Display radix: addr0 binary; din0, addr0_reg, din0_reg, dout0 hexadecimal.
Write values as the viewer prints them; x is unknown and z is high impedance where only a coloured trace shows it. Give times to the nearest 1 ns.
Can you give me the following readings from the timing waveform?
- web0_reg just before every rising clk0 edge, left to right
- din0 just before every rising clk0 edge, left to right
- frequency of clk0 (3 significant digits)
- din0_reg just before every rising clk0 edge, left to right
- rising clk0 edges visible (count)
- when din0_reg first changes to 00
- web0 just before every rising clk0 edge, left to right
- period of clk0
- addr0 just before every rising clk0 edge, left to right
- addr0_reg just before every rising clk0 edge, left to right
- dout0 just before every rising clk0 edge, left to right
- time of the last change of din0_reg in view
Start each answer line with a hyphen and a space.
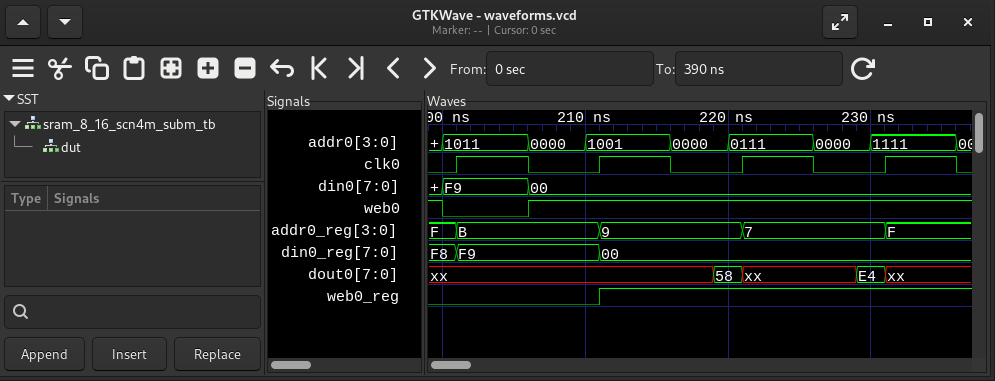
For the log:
- 0 0 1 1
- F9, 00, 00, 00
- 100 MHz
- F8, F9, 00, 00
- 4
- 211 ns
- 0 1 1 1
- 10 ns
- 1011, 1001, 0111, 1111
- F, B, 9, 7
- xx, xx, 58, E4
- 211 ns
